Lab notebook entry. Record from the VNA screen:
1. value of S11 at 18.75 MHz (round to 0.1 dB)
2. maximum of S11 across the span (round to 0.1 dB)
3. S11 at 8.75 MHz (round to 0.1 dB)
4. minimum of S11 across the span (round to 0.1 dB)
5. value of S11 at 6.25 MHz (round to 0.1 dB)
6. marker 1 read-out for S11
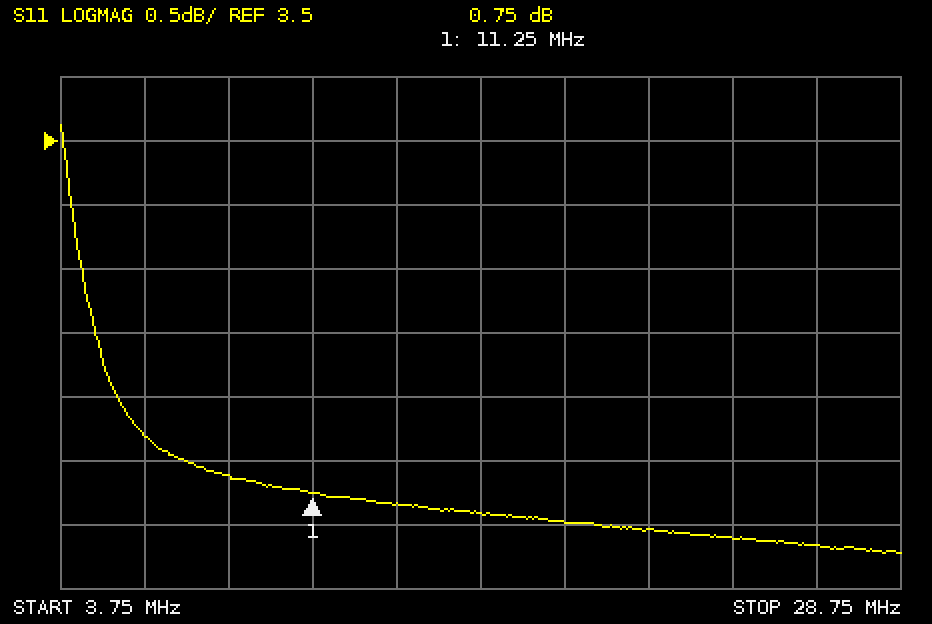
0.5 dB
3.6 dB
0.9 dB
0.3 dB
1.2 dB
0.75 dB
